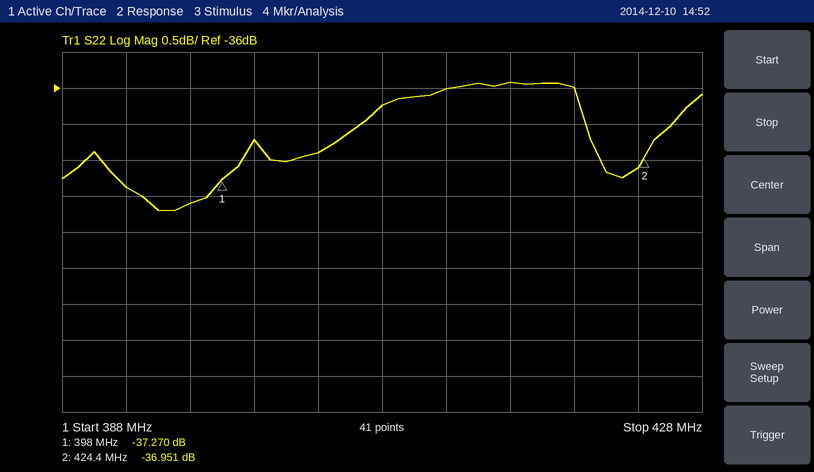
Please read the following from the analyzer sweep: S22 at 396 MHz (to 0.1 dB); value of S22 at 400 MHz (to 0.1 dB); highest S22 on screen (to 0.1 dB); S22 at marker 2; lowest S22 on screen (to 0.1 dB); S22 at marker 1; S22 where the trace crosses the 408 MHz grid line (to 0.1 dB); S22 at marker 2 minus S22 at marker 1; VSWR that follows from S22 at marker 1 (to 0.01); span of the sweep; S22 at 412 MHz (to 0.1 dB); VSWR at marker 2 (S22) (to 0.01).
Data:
-37.6 dB
-36.7 dB
-35.9 dB
-36.951 dB
-37.7 dB
-37.270 dB
-36.2 dB
0.319 dB
1.03
40 MHz
-36.0 dB
1.03
